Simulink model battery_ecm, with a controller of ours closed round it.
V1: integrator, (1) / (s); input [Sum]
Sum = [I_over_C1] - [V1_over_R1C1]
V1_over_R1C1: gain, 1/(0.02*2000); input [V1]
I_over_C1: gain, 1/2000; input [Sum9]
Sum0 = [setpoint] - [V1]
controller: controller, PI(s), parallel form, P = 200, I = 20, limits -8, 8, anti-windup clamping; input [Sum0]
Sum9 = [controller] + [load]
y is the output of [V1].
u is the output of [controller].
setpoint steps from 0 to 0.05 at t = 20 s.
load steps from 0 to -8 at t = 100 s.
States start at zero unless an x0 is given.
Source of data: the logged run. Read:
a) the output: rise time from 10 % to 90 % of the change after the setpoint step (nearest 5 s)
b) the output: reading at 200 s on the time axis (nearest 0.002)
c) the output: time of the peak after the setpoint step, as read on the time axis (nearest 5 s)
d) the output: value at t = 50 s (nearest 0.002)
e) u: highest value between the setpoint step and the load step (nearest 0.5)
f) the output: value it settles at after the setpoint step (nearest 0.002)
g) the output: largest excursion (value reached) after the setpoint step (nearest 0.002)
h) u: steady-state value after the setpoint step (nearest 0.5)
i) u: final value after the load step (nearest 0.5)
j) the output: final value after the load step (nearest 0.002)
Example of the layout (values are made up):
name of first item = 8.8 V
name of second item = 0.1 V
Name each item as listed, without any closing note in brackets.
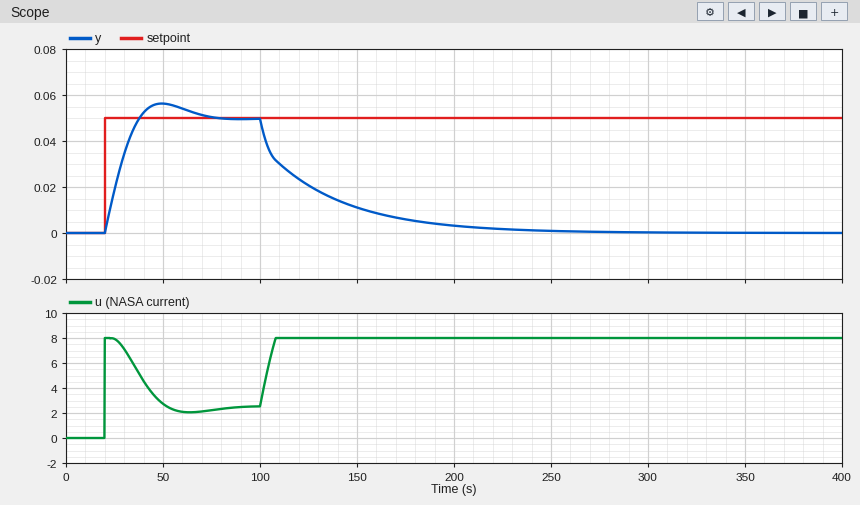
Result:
the output: rise time from 10 % to 90 % of the change after the setpoint step = 15 s
the output: reading at 200 s on the time axis = 0.004
the output: time of the peak after the setpoint step, as read on the time axis = 50 s
the output: value at t = 50 s = 0.056
u: highest value between the setpoint step and the load step = 8.0
the output: value it settles at after the setpoint step = 0.050
the output: largest excursion (value reached) after the setpoint step = 0.056
u: steady-state value after the setpoint step = 2.5
u: final value after the load step = 8.0
the output: final value after the load step = 0.000
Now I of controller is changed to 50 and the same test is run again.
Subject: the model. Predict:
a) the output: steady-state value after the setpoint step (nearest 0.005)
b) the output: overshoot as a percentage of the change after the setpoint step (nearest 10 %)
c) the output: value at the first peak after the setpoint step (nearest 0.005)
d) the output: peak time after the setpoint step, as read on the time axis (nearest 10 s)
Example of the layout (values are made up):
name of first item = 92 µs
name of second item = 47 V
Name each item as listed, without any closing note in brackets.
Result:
the output: steady-state value after the setpoint step = 0.050
the output: overshoot as a percentage of the change after the setpoint step = 20 %
the output: value at the first peak after the setpoint step = 0.060
the output: peak time after the setpoint step, as read on the time axis = 40 s
